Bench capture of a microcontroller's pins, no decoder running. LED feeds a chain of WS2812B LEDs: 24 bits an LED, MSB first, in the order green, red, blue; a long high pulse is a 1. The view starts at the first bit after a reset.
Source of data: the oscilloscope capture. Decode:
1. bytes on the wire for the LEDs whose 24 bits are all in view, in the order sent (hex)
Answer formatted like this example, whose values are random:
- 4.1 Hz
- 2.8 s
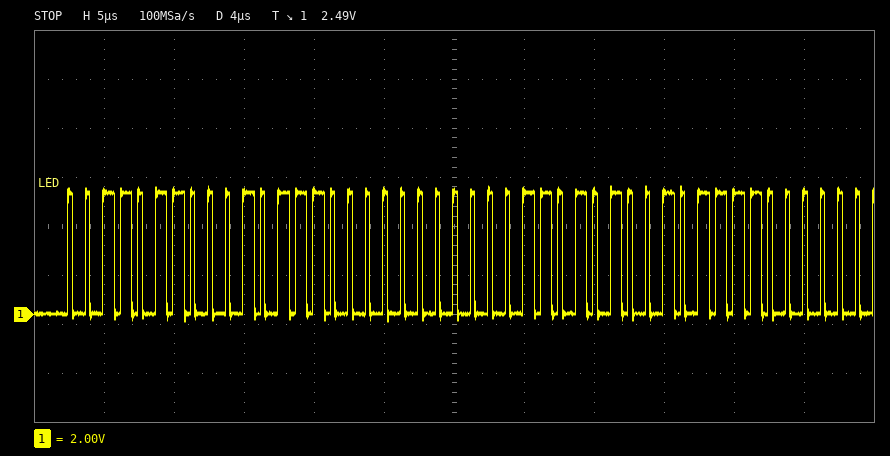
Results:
- 36 2E 00
